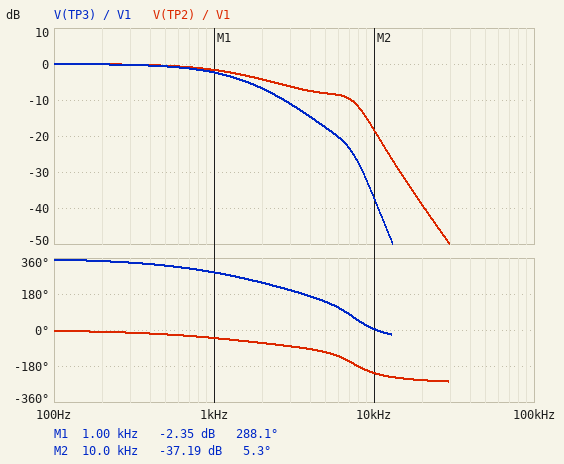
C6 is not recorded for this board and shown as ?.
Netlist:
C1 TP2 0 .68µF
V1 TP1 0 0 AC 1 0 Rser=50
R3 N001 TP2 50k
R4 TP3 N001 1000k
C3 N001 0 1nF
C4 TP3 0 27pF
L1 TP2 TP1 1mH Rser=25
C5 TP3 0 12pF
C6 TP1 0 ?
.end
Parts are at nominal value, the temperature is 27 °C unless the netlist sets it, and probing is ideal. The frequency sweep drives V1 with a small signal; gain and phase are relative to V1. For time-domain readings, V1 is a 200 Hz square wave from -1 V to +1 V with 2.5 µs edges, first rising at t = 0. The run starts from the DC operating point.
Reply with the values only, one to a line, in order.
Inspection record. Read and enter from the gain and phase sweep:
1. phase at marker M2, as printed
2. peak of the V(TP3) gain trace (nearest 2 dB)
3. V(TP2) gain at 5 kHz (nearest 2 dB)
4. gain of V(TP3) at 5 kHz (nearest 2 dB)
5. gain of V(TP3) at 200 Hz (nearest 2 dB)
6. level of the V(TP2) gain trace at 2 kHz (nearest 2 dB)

5.3 deg
0 dB
-8 dB
-18 dB
0 dB
-4 dB
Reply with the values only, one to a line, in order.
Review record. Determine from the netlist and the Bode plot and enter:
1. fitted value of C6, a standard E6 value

1.5 µF
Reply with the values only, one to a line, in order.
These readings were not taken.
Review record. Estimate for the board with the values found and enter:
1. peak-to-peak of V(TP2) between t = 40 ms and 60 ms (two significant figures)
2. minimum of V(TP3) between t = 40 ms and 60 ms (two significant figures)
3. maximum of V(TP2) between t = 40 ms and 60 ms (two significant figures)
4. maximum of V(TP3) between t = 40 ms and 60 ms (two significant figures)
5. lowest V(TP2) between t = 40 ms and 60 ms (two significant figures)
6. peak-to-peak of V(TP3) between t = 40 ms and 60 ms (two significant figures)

2.0 V
-1.0 V
1.0 V
1.0 V
-1.0 V
2.0 V
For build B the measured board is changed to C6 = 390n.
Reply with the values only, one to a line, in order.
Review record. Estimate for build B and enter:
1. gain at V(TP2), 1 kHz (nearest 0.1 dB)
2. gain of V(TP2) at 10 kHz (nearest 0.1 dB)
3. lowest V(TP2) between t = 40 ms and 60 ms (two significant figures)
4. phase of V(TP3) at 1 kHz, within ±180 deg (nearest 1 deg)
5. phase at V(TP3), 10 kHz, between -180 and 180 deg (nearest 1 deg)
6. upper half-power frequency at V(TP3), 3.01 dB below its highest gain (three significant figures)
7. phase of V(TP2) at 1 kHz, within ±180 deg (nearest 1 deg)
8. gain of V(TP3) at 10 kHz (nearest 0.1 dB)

-0.5 dB
-10.1 dB
-1.0 V
-56 deg
61 deg
1.66 kHz
-25 deg
-29.0 dB
